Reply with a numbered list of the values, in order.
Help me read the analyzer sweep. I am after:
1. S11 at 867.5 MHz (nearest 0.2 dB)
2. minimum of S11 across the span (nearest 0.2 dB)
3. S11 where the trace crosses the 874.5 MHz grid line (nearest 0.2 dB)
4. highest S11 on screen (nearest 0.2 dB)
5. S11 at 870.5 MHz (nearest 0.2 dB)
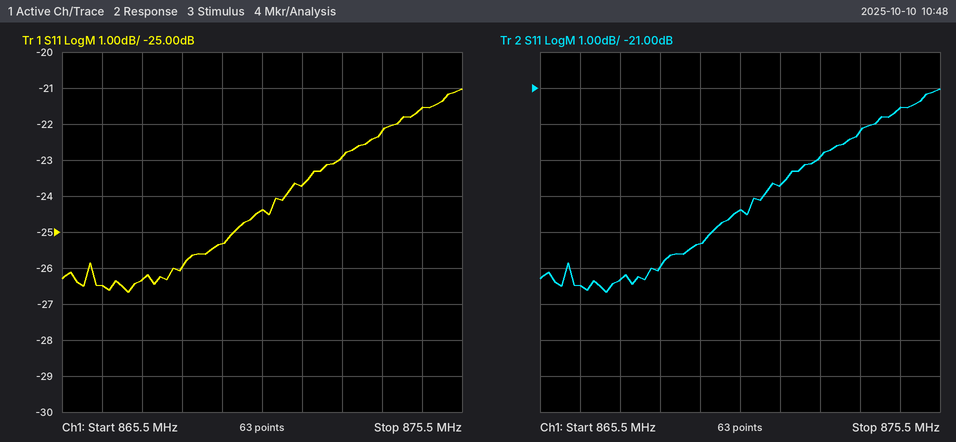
1. -26.4 dB
2. -26.6 dB
3. -21.6 dB
4. -21.0 dB
5. -24.4 dB
